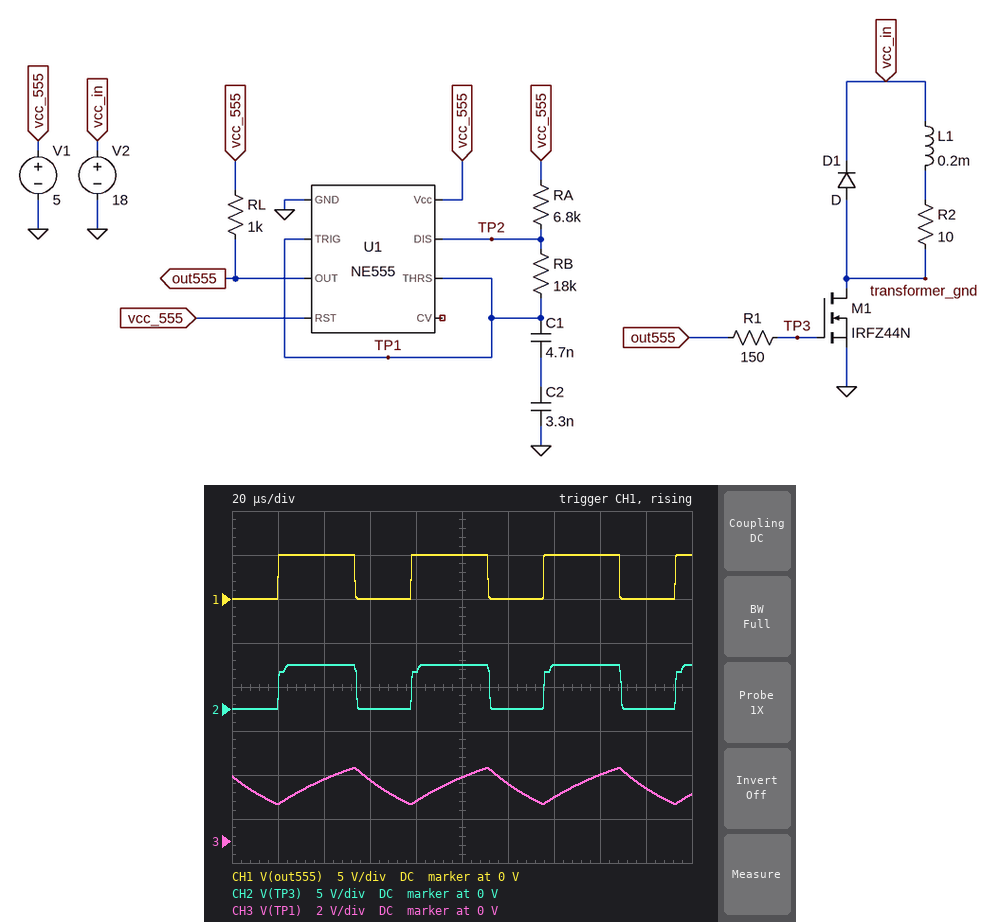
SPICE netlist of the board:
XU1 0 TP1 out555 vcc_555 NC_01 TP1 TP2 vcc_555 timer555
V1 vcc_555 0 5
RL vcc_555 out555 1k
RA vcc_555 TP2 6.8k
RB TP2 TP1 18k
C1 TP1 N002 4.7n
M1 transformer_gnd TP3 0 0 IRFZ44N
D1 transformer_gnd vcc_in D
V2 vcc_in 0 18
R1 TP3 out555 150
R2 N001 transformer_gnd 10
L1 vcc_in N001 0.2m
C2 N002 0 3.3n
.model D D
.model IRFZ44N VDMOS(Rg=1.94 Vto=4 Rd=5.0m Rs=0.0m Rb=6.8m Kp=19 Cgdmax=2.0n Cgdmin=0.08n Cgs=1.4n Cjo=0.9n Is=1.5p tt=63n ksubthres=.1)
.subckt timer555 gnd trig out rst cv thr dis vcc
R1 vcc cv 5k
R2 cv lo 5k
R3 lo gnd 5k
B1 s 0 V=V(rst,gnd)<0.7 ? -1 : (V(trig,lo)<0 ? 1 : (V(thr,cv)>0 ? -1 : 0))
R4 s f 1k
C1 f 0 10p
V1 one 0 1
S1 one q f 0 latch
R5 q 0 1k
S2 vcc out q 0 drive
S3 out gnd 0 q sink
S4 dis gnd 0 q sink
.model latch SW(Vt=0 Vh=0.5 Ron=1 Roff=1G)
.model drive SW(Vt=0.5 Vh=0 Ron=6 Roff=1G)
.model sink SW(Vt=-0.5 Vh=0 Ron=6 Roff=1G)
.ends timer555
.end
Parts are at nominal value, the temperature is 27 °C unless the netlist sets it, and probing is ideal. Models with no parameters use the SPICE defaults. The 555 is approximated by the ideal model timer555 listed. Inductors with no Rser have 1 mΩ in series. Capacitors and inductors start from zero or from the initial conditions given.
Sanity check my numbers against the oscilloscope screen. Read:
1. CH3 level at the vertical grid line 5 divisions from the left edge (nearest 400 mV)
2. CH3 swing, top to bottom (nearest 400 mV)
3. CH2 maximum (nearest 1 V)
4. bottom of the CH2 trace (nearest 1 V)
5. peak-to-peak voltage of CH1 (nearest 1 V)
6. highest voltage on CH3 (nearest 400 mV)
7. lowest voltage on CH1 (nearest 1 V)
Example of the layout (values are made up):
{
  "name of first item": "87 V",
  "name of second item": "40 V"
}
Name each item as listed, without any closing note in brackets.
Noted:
{
  "CH3 level at the vertical grid line 5 divisions from the left edge": "2.8 V",
  "CH3 swing, top to bottom": "1.6 V",
  "CH2 maximum": "5 V",
  "bottom of the CH2 trace": "0 V",
  "peak-to-peak voltage of CH1": "5 V",
  "highest voltage on CH3": "3.2 V",
  "lowest voltage on CH1": "0 V"
}
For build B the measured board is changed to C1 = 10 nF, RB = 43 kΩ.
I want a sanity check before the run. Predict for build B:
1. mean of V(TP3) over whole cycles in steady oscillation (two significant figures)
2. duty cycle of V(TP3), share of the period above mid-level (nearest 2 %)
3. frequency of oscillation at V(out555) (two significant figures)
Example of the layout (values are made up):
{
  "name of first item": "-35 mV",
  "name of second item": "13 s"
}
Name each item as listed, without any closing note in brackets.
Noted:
{
  "mean of V(TP3) over whole cycles in steady oscillation": "2.7 V",
  "duty cycle of V(TP3), share of the period above mid-level": "54 %",
  "frequency of oscillation at V(out555)": "6.3 kHz"
}
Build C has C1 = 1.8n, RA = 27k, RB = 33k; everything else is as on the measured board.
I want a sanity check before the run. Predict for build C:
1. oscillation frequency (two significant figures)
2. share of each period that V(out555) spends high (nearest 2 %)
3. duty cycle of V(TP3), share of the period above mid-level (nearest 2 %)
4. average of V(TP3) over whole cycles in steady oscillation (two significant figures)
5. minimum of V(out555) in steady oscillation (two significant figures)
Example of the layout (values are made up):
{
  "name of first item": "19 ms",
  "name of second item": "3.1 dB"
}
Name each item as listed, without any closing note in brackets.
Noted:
{
  "oscillation frequency": "13 kHz",
  "share of each period that V(out555) spends high": "64 %",
  "duty cycle of V(TP3), share of the period above mid-level": "66 %",
  "average of V(TP3) over whole cycles in steady oscillation": "3.2 V",
  "minimum of V(out555) in steady oscillation": "30 mV"
}
